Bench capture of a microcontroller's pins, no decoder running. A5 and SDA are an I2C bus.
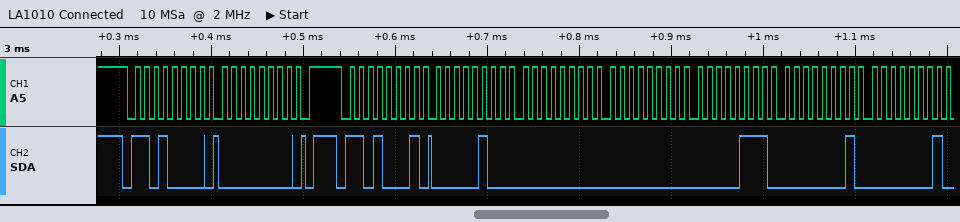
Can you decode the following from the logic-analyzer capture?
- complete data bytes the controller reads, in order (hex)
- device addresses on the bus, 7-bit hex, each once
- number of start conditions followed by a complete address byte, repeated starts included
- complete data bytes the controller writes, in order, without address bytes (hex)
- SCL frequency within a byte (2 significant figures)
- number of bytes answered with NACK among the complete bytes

04 00 00 07 01 01
0x68
2
00
100 kHz
0
